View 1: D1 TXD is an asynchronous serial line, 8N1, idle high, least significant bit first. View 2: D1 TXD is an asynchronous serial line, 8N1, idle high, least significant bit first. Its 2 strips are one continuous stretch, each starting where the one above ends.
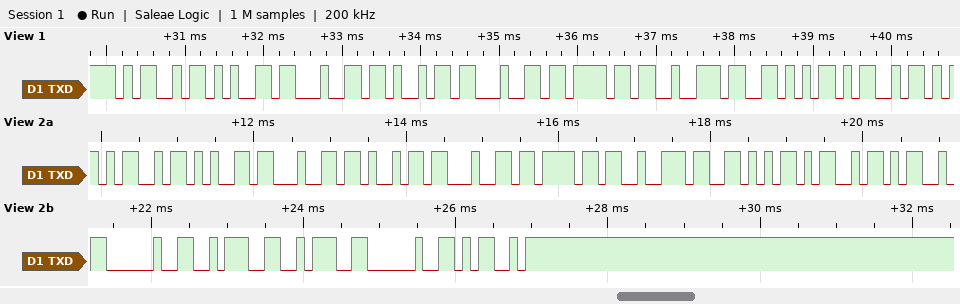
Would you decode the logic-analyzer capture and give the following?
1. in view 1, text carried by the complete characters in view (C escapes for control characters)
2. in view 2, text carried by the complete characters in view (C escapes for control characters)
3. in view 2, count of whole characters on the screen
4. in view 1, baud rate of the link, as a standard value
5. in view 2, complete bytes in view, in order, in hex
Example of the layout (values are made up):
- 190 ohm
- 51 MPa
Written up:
- "MedidorVM"
- "MedidorVMM :: M"
- 15
- 9600 baud
- 0x4D 0x65 0x64 0x69 0x64 0x6F 0x72 0x56 0x4D 0x4D 0x20 0x3A 0x3A 0x20 0x4D
